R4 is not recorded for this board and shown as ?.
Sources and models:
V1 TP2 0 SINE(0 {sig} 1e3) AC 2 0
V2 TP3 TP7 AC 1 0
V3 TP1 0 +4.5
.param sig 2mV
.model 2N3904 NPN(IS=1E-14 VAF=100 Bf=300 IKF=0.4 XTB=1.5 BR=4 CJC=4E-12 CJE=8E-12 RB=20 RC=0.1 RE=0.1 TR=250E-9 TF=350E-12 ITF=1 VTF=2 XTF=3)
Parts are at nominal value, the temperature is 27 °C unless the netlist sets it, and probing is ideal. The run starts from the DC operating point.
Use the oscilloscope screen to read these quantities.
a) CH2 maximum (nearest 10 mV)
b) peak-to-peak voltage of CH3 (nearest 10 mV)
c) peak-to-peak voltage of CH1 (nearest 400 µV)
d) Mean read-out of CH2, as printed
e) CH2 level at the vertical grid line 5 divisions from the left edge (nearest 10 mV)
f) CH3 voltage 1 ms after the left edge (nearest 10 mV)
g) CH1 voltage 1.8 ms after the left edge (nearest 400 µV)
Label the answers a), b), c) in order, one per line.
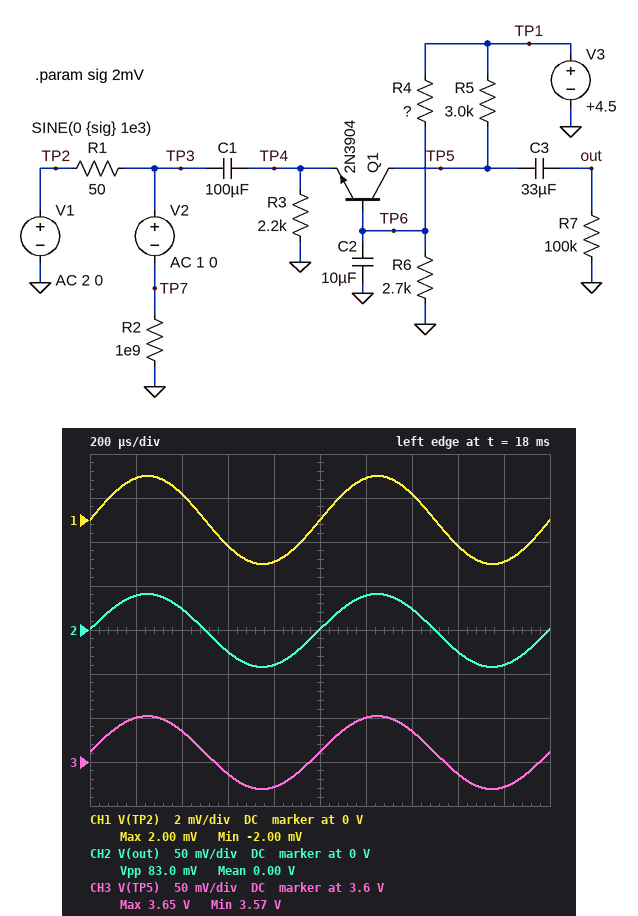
a) 40 mV
b) 80 mV
c) 4.0 mV
d) 0.00 V
e) 0 V
f) 3.61 V
g) -2.0 mV
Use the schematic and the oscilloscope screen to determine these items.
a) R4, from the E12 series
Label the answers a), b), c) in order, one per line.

a) 6.8 kΩ
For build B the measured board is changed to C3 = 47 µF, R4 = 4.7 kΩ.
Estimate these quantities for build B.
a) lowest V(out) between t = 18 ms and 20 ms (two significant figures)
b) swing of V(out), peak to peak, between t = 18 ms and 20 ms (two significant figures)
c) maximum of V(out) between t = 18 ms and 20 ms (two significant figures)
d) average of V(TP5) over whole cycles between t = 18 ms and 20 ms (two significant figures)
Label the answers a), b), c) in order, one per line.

a) -54 mV
b) 110 mV
c) 53 mV
d) 3.1 V
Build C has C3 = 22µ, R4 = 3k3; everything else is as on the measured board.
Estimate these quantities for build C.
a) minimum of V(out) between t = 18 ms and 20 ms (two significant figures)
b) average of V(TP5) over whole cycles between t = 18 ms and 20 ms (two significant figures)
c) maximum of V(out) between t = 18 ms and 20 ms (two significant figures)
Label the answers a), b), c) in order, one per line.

a) -63 mV
b) 2.6 V
c) 62 mV
